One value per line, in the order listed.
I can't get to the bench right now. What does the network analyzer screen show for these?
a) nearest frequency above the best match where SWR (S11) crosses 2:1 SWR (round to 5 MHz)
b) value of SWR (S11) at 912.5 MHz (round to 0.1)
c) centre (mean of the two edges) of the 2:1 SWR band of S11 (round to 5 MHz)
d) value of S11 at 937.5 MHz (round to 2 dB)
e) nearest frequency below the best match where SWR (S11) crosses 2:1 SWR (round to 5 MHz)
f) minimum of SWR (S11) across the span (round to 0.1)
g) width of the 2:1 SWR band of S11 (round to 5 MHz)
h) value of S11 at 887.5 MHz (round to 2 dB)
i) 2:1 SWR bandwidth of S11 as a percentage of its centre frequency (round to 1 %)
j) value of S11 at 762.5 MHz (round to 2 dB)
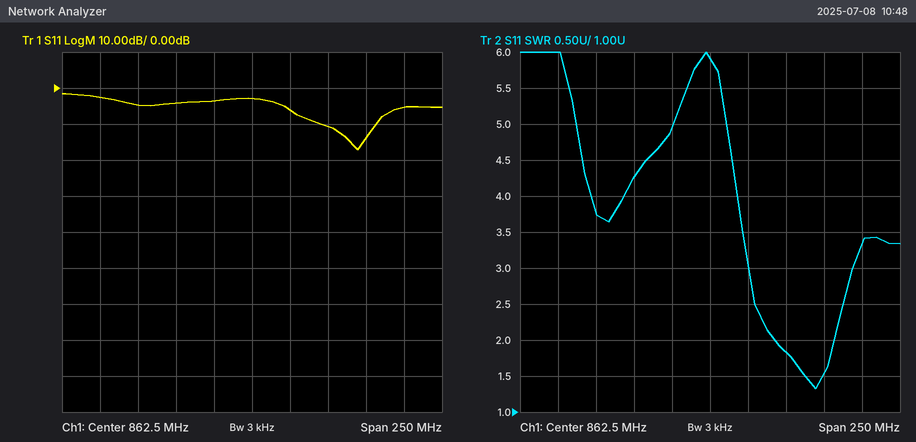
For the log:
945 MHz
1.8
925 MHz
-14 dB
905 MHz
1.3
40 MHz
-6 dB
4 %
-2 dB
